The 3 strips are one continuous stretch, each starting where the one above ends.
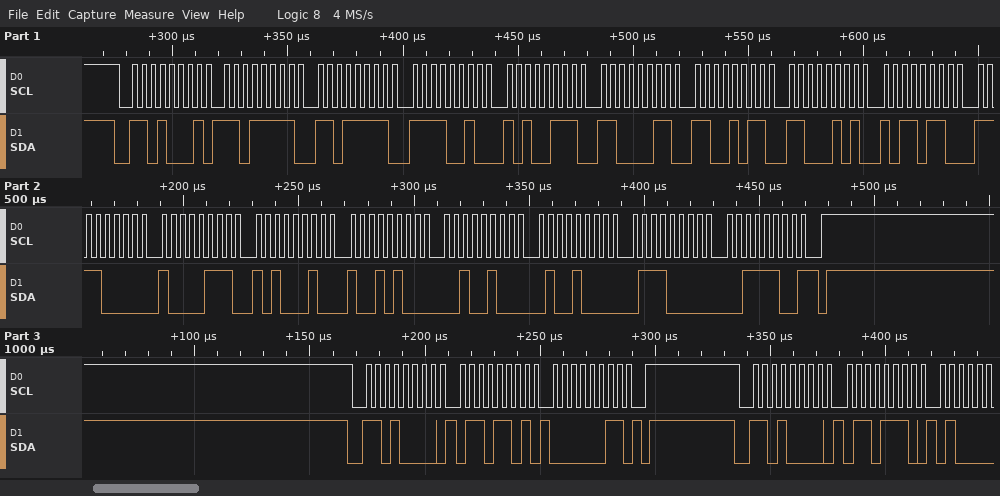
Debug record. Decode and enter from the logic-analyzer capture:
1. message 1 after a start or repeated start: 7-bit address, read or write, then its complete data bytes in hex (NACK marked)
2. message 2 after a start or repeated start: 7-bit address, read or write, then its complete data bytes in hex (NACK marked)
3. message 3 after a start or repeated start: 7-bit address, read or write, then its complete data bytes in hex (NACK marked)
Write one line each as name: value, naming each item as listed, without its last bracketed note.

message 1 after a start or repeated start: 7-bit address, read or write, then its complete data bytes in hex: 0x68 read: DF DF F2 A7 C3 CB C5 B6 F0 87 A2 94 24 48 70 3C NACK
message 2 after a start or repeated start: 7-bit address, read or write, then its complete data bytes in hex: 0x68 write: 6D 03
message 3 after a start or repeated start: 7-bit address, read or write, then its complete data bytes in hex: 0x68 write: 6E
